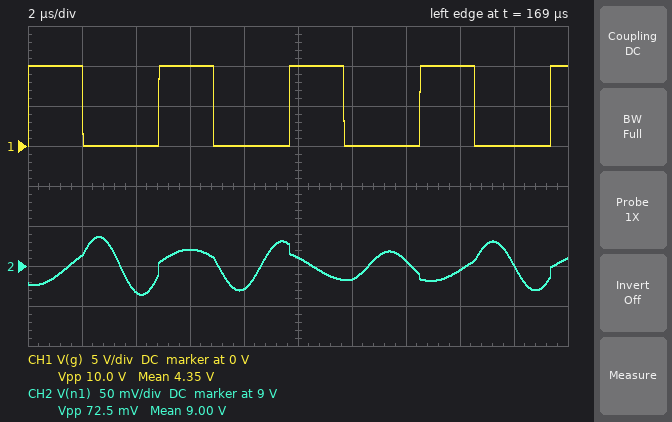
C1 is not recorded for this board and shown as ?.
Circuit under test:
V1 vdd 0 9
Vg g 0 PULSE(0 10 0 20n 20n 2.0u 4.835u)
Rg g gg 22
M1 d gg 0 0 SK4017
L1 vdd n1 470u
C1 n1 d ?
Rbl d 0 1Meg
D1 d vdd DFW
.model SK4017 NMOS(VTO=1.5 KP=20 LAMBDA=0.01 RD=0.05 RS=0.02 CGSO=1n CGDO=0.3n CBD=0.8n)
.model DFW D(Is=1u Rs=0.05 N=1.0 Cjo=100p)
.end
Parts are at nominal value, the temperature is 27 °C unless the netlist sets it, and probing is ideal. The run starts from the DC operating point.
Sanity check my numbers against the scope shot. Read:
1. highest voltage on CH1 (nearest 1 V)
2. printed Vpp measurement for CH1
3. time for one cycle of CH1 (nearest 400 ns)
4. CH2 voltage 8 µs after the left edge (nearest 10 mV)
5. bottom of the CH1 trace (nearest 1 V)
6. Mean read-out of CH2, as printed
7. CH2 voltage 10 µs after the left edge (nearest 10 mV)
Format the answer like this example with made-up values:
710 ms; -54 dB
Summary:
10 V; 10.0 V; 4.8 µs; 8.97 V; 0 V; 9.00 V; 9.01 V
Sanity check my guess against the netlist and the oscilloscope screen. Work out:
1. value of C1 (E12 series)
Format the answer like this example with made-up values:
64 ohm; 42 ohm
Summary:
1.5 nF
